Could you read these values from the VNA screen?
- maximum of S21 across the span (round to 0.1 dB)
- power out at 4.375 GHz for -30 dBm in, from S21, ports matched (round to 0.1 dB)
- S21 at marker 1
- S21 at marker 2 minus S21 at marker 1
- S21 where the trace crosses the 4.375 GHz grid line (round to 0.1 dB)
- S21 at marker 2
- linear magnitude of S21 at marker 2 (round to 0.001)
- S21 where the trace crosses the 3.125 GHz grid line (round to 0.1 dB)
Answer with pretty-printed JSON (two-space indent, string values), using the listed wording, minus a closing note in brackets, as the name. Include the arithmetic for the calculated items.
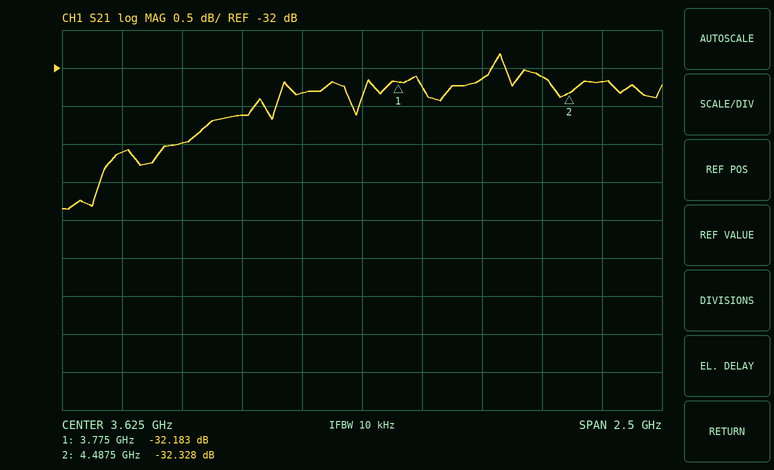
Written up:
{
  "maximum of S21 across the span": "-31.8 dB",
  "power out at 4.375 GHz for -30 dBm in, from S21, ports matched": "-30 dBm + (-32.1 dB) = -62.1 dBm",
  "S21 at marker 1": "-32.183 dB",
  "S21 at marker 2 minus S21 at marker 1": "-32.328 − (-32.183) = -0.145 dB",
  "S21 where the trace crosses the 4.375 GHz grid line": "-32.1 dB",
  "S21 at marker 2": "-32.328 dB",
  "linear magnitude of S21 at marker 2": "10^(-32.328/20) ≈ 0.024",
  "S21 where the trace crosses the 3.125 GHz grid line": "-32.6 dB"
}
